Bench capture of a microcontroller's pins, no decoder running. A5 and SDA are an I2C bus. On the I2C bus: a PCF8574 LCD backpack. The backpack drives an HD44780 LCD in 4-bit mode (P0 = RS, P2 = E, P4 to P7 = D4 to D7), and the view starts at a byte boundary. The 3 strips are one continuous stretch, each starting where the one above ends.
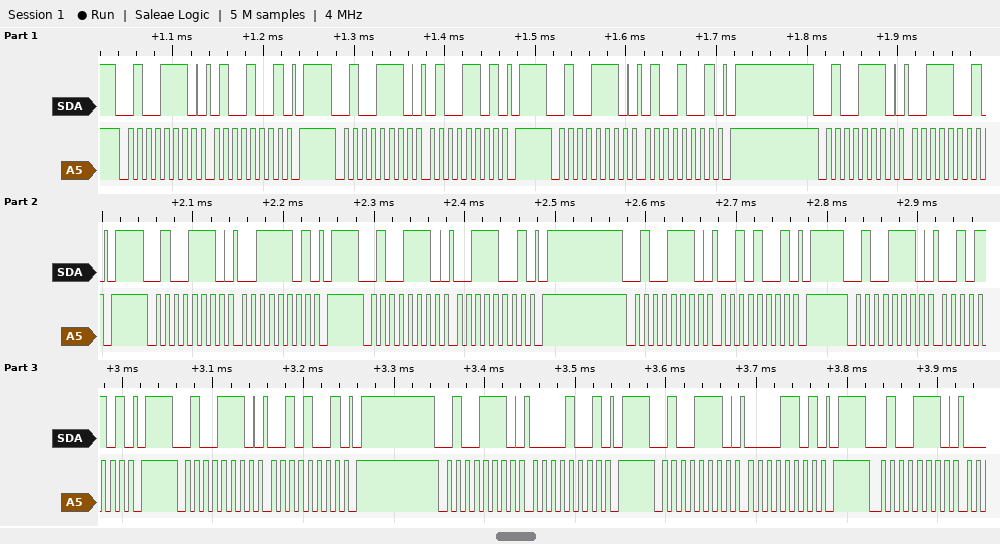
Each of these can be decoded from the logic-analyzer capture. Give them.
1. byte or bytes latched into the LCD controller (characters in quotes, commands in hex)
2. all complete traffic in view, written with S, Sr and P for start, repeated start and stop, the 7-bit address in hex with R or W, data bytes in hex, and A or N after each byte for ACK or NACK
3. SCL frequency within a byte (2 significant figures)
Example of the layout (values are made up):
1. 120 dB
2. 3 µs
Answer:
1. 'C'
2. S 27W A 49 A P S 27W A 4D A P S 27W A 49 A P S 27W A 39 A P S 27W A 3D A P S 27W A 39 A P S 27W A 29 A P S 27W A 2D A P S 27W A 29 A P S 27W A 09 A P S 27W A 0D A P S 27W A
3. 100 kHz
